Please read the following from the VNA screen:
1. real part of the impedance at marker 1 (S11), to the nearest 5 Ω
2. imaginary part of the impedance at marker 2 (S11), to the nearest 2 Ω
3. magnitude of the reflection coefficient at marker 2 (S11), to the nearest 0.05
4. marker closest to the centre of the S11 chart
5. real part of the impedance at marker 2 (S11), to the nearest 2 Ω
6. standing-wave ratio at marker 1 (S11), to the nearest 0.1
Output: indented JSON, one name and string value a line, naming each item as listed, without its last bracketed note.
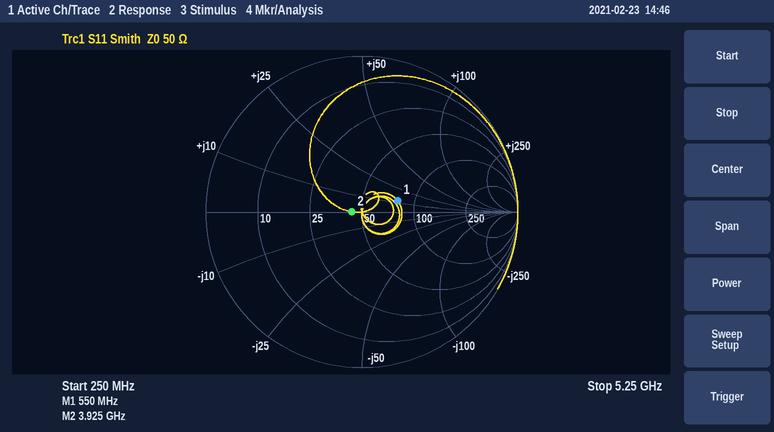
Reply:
{
  "real part of the impedance at marker 1 (S11), to the nearest 5 Ω": "80 Ω",
  "imaginary part of the impedance at marker 2 (S11), to the nearest 2 Ω": "0 Ω",
  "magnitude of the reflection coefficient at marker 2 (S11), to the nearest 0.05": "0.05",
  "marker closest to the centre of the S11 chart": "marker 2",
  "real part of the impedance at marker 2 (S11), to the nearest 2 Ω": "44 Ω",
  "standing-wave ratio at marker 1 (S11), to the nearest 0.1": "1.6"
}
